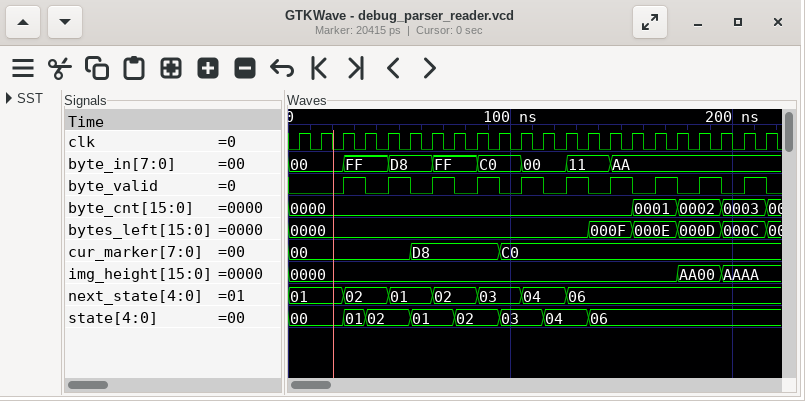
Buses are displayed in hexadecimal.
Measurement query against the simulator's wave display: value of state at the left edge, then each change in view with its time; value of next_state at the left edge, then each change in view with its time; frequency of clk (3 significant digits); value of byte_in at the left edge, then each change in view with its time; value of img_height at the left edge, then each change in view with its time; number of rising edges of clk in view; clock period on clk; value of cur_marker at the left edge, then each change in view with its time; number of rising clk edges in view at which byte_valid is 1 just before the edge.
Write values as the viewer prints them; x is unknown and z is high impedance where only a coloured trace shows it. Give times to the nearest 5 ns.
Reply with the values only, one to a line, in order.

00, 01 at 25 ns, 02 at 35 ns, 01 at 55 ns, 02 at 75 ns, 03 at 95 ns, 04 at 115 ns, 06 at 135 ns
01, 02 at 25 ns, 01 at 45 ns, 02 at 65 ns, 03 at 85 ns, 04 at 105 ns, 06 at 125 ns
100 MHz
00, FF at 25 ns, D8 at 45 ns, FF at 65 ns, C0 at 85 ns, 00 at 105 ns, 11 at 125 ns, AA at 145 ns
0000, AA00 at 175 ns, AAAA at 195 ns
22
10 ns
00, D8 at 55 ns, C0 at 95 ns
10
